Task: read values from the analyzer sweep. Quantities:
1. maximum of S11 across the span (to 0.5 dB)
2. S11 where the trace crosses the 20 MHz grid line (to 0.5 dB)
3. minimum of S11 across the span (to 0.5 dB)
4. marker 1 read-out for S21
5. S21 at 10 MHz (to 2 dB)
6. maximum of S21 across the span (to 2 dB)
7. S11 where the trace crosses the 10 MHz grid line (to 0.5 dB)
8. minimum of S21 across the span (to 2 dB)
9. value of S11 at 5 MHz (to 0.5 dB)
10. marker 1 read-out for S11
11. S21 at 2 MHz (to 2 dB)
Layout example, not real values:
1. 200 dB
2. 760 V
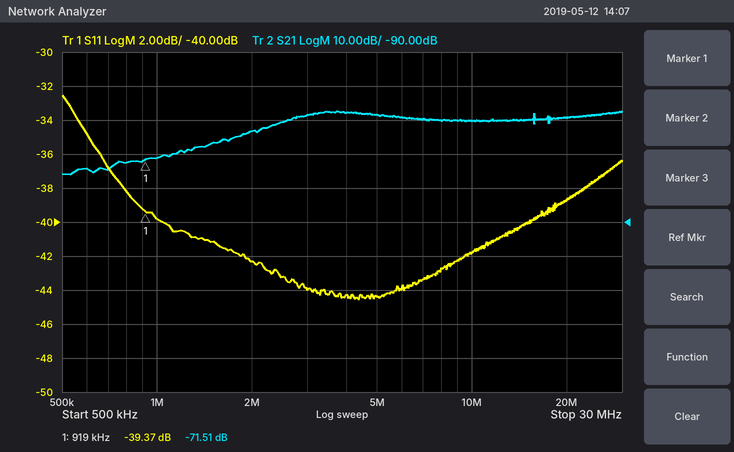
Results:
1. -32.5 dB
2. -38.5 dB
3. -44.5 dB
4. -71.51 dB
5. -60 dB
6. -58 dB
7. -42.0 dB
8. -76 dB
9. -44.5 dB
10. -39.37 dB
11. -64 dB
